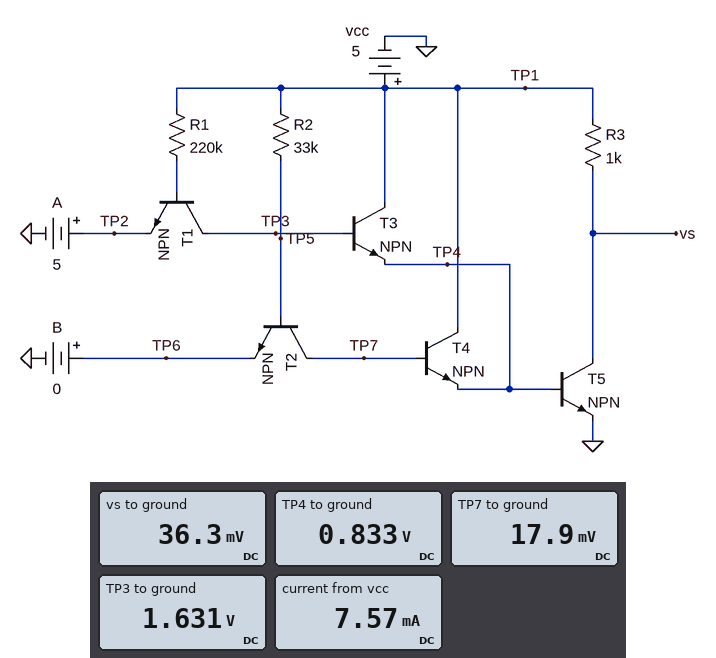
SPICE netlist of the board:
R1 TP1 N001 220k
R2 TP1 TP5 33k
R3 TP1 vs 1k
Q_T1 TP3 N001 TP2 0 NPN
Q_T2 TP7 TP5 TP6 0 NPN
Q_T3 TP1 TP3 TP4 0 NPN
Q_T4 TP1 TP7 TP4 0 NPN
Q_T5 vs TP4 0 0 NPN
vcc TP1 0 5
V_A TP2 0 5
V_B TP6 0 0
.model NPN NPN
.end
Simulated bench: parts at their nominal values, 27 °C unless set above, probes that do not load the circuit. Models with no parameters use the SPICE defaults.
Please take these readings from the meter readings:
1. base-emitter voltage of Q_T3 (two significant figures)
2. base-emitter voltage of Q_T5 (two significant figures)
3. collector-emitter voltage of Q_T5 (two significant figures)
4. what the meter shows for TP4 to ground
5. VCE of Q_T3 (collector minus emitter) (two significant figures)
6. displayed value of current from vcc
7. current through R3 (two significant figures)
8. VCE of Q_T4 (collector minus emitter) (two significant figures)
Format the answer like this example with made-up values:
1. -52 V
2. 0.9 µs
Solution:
1. 800 mV
2. 830 mV
3. 36 mV
4. 0.833 V
5. 4.2 V
6. 7.57 mA
7. 5.0 mA
8. 4.2 V
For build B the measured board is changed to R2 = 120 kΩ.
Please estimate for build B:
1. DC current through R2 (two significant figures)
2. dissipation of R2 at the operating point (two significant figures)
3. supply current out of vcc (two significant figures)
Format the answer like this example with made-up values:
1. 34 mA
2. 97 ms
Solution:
1. 36 µA
2. 150 µW
3. 7.5 mA
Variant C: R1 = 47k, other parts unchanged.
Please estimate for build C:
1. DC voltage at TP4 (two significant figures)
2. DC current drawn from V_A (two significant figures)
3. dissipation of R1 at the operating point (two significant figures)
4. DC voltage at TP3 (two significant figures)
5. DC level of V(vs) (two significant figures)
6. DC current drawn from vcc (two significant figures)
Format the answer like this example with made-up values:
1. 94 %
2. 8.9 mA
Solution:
1. 860 mV
2. 55 µA
3. 140 µW
4. 1.7 V
5. 23 mV
6. 16 mA
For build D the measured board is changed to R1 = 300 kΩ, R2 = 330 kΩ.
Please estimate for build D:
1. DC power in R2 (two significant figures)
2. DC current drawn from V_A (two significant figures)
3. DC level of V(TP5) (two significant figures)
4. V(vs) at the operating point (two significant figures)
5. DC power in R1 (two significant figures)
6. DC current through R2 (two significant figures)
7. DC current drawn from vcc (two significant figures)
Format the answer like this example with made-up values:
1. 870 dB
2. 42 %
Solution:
1. 57 µW
2. 9.1 µA
3. 680 mV
4. 41 mV
5. 25 µW
6. 13 µA
7. 6.8 mA
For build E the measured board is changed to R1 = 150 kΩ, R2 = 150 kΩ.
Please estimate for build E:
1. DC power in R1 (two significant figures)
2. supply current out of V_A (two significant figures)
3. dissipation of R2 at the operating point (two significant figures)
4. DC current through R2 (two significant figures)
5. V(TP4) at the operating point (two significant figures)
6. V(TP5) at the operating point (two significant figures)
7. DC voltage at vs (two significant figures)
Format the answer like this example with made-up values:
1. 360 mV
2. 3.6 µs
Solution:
1. 48 µW
2. 18 µA
3. 120 µW
4. 29 µA
5. 840 mV
6. 700 mV
7. 32 mV
